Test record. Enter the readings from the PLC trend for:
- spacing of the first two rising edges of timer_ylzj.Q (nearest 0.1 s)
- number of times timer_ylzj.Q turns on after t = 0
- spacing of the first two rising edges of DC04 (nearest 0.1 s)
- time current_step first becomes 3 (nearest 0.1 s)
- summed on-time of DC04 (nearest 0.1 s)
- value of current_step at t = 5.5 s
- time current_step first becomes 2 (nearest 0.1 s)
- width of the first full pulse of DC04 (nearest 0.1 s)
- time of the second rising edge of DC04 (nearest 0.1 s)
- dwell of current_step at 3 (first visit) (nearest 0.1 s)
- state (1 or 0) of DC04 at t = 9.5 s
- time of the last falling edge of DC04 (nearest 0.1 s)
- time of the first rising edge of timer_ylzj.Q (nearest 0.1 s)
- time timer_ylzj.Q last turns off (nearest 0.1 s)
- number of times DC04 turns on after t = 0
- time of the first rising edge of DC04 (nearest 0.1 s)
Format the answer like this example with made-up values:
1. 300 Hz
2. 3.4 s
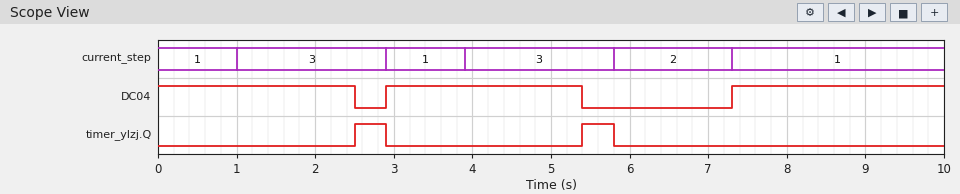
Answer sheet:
1. 2.9 s
2. 2
3. 4.4 s
4. 1.0 s
5. 7.7 s
6. 3
7. 5.8 s
8. 2.5 s
9. 7.3 s
10. 1.9 s
11. 1
12. 5.4 s
13. 2.5 s
14. 5.8 s
15. 2
16. 2.9 s
